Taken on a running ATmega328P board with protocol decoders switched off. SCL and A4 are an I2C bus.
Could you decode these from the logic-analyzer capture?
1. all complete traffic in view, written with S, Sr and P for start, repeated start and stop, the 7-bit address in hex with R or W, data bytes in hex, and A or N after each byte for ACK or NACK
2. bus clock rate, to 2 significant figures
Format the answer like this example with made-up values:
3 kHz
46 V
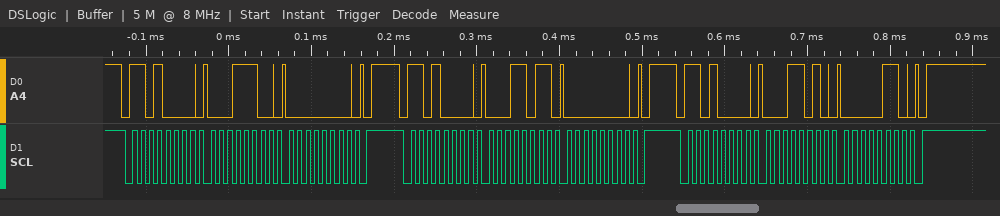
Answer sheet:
S 68W A 1C A 00 A P S 68W A 1B A 00 A P S 68W A 1A A 06 A P
100 kHz
